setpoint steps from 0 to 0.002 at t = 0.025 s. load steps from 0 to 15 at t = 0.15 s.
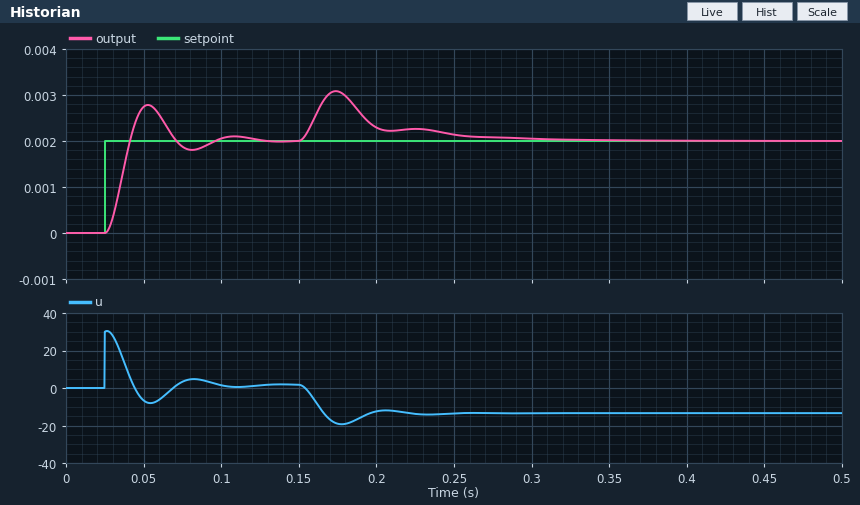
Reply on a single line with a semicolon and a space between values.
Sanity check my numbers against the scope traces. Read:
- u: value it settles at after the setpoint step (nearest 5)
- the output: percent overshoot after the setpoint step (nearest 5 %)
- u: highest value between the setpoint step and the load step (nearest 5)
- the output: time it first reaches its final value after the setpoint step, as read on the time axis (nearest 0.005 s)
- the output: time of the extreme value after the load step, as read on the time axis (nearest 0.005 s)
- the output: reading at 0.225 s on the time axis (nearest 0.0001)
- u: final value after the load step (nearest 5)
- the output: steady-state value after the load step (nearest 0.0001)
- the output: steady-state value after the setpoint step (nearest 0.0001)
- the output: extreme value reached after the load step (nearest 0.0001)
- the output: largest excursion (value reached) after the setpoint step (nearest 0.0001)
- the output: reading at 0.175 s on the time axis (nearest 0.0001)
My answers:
0; 40 %; 30; 0.040 s; 0.175 s; 0.0023; -15; 0.0020; 0.0020; 0.0031; 0.0028; 0.0031
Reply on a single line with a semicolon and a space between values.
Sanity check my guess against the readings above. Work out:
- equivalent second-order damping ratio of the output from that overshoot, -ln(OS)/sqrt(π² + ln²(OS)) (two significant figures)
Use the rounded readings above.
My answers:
0.28
